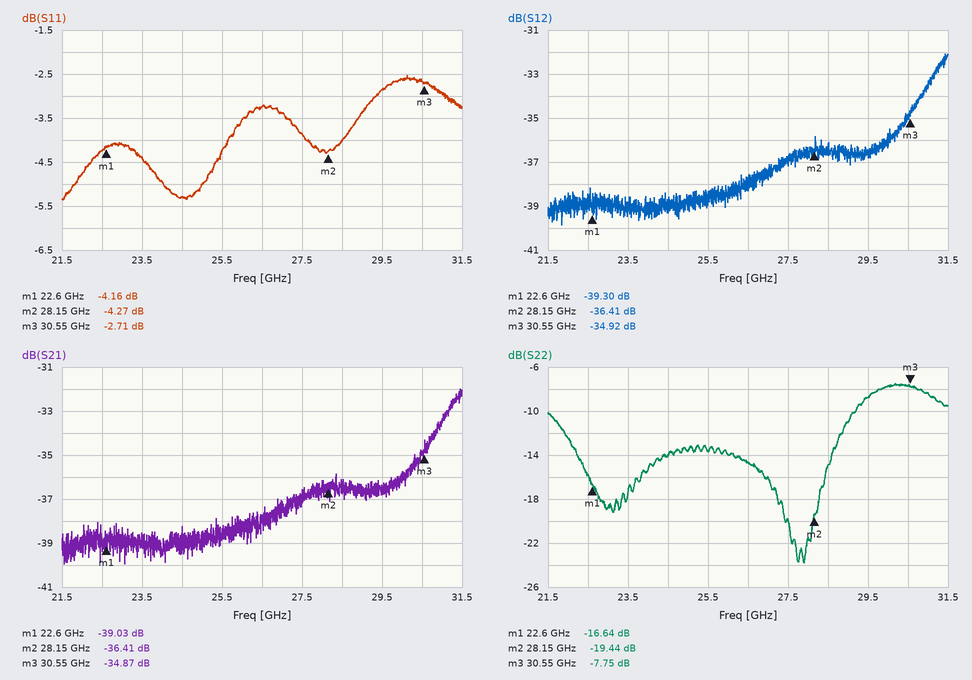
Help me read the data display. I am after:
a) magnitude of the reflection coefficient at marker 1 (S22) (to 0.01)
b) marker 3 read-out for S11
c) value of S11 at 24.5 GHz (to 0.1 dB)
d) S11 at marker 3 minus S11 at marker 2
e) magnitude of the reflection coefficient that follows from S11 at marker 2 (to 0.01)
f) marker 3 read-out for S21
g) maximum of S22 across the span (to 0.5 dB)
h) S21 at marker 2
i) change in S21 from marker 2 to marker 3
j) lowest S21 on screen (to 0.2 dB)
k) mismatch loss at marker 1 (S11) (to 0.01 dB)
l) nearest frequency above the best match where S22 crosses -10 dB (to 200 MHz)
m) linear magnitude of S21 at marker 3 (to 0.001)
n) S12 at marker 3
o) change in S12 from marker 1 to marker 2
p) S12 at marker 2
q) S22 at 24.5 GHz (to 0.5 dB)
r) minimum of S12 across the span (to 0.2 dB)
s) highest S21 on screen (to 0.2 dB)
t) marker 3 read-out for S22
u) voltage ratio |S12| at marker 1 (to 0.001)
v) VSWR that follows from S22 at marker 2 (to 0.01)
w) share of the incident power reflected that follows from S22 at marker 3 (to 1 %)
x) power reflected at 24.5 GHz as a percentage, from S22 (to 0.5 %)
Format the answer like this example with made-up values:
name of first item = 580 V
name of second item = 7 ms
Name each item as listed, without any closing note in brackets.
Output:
magnitude of the reflection coefficient at marker 1 (S22) = 0.15
marker 3 read-out for S11 = -2.71 dB
value of S11 at 24.5 GHz = -5.3 dB
S11 at marker 3 minus S11 at marker 2 = 1.56 dB
magnitude of the reflection coefficient that follows from S11 at marker 2 = 0.61
marker 3 read-out for S21 = -34.87 dB
maximum of S22 across the span = -7.5 dB
S21 at marker 2 = -36.41 dB
change in S21 from marker 2 to marker 3 = 1.54 dB
lowest S21 on screen = -40.0 dB
mismatch loss at marker 1 (S11) = 2.10 dB
nearest frequency above the best match where S22 crosses -10 dB = 29.2 GHz
linear magnitude of S21 at marker 3 = 0.018
S12 at marker 3 = -34.92 dB
change in S12 from marker 1 to marker 2 = 2.89 dB
S12 at marker 2 = -36.41 dB
S22 at 24.5 GHz = -14.0 dB
minimum of S12 across the span = -39.8 dB
highest S21 on screen = -32.0 dB
marker 3 read-out for S22 = -7.75 dB
voltage ratio |S12| at marker 1 = 0.011
VSWR that follows from S22 at marker 2 = 1.24
share of the incident power reflected that follows from S22 at marker 3 = 17 %
power reflected at 24.5 GHz as a percentage, from S22 = 4.0 %
